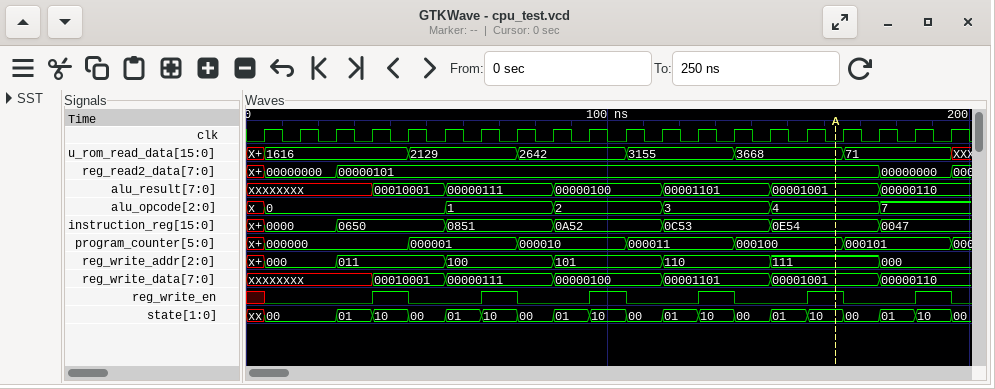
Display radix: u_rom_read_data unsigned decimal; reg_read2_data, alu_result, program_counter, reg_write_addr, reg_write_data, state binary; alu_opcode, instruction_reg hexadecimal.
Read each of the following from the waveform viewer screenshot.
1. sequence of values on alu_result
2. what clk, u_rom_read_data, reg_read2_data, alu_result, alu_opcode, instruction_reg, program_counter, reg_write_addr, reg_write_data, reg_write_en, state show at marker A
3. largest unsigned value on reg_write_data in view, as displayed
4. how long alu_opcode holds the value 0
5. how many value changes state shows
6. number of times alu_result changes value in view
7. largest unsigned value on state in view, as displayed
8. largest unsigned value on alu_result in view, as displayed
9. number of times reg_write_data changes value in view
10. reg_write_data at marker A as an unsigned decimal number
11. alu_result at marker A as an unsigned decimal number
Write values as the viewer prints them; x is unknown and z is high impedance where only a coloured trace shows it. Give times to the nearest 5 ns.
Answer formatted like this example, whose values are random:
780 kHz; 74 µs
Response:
xxxxxxxx, 00010001, 00000111, 00000100, 00001101, 00001001, 00000110; clk=0, u_rom_read_data=3668, reg_read2_data=00000101, alu_result=00001001, alu_opcode=4, instruction_reg=0E54, program_counter=000100, reg_write_addr=111, reg_write_data=00001001, reg_write_en=1, state=10; 00010001; 50 ns; 19; 6; 10; 00010001; 6; 9; 9
